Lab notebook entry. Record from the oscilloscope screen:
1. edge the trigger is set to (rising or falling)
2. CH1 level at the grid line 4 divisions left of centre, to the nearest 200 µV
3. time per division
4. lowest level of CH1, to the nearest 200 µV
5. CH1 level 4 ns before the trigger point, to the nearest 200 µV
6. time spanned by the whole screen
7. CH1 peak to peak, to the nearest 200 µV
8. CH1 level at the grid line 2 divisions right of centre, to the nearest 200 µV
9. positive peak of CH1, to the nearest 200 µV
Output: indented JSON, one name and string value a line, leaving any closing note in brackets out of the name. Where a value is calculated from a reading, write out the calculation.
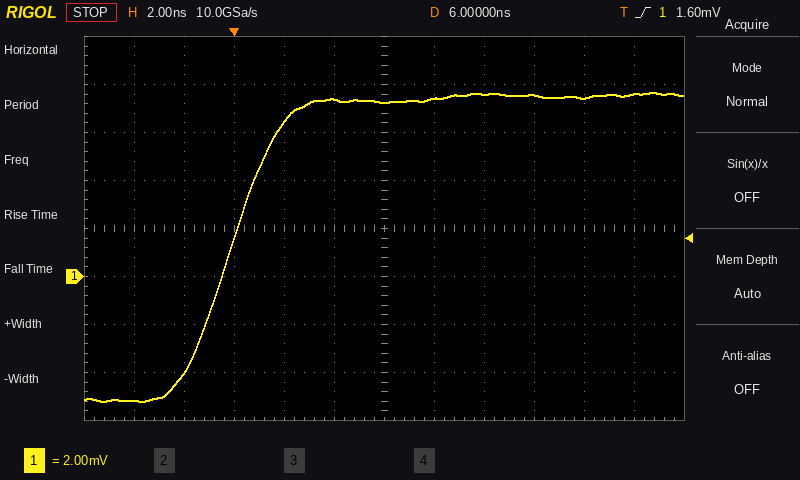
{
  "edge the trigger is set to": "rising",
  "CH1 level at the grid line 4 divisions left of centre, to the nearest 200 µV": "-4.0 mV",
  "time per division": "2 ns",
  "lowest level of CH1, to the nearest 200 µV": "-5.2 mV",
  "CH1 level 4 ns before the trigger point, to the nearest 200 µV": "-5.2 mV",
  "time spanned by the whole screen": "24 ns",
  "CH1 peak to peak, to the nearest 200 µV": "7.6 mV − (-5.2 mV) = 12.8 mV",
  "CH1 level at the grid line 2 divisions right of centre, to the nearest 200 µV": "7.6 mV",
  "positive peak of CH1, to the nearest 200 µV": "7.6 mV"
}
